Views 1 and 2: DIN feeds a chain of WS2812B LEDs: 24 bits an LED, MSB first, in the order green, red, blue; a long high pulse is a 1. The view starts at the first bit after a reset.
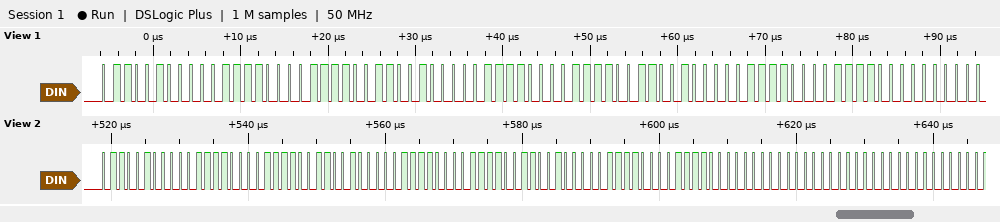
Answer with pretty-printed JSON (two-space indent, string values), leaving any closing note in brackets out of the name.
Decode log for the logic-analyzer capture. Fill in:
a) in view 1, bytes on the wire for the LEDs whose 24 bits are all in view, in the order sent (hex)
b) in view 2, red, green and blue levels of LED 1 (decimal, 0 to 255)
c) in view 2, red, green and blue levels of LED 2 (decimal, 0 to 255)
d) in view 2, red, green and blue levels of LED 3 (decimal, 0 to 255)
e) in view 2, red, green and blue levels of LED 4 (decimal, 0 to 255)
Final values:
{
  "in view 1, bytes on the wire for the LEDs whose 24 bits are all in view, in the order sent": "64 1E 1E 64 1E 1E 64 1E 1E",
  "in view 2, red, green and blue levels of LED 1": "30, 100, 30",
  "in view 2, red, green and blue levels of LED 2": "30, 100, 30",
  "in view 2, red, green and blue levels of LED 3": "30, 100, 30",
  "in view 2, red, green and blue levels of LED 4": "0, 0, 0"
}
